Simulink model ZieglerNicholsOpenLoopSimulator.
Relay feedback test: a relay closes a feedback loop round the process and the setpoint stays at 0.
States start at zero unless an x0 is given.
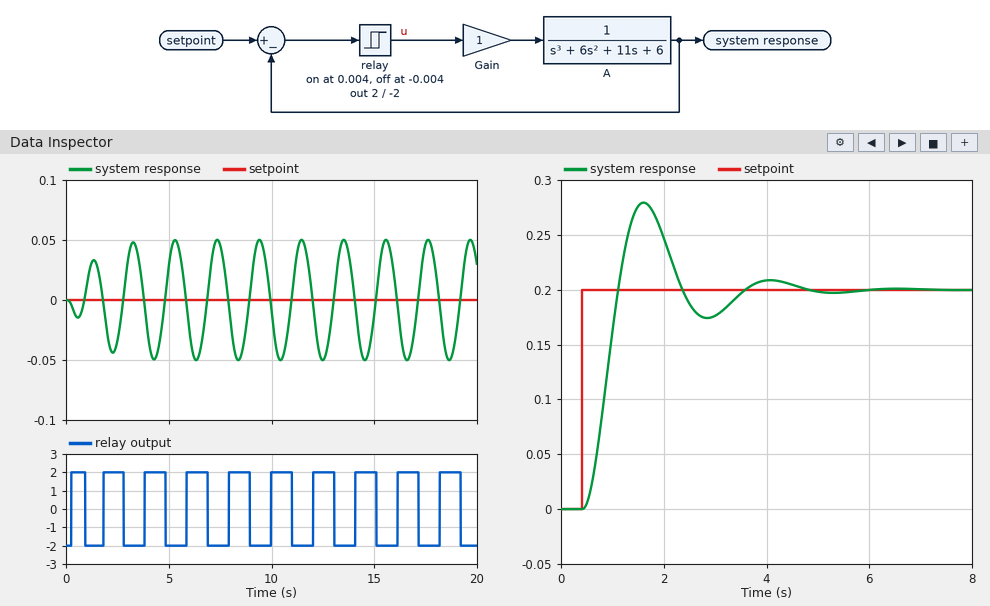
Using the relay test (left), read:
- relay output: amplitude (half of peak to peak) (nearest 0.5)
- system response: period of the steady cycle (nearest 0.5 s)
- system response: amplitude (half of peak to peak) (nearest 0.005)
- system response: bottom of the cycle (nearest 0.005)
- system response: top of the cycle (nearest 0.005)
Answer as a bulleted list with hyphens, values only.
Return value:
- 2.0
- 2.0 s
- 0.050
- -0.050
- 0.050
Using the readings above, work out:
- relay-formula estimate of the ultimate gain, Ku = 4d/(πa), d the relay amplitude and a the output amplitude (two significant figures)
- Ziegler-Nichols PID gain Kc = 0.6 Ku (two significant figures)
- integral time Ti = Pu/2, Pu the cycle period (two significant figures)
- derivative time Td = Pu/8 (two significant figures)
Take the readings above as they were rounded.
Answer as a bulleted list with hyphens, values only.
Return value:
- 51
- 31
- 1.0 s
- 0.25 s
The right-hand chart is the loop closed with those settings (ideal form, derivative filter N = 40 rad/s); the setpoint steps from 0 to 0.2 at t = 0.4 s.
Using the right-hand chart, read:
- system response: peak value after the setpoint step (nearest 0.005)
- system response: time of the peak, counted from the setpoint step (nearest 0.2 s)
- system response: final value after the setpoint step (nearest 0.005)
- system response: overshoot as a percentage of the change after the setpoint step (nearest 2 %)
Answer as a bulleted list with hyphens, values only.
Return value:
- 0.280
- 1.2 s
- 0.200
- 40 %
